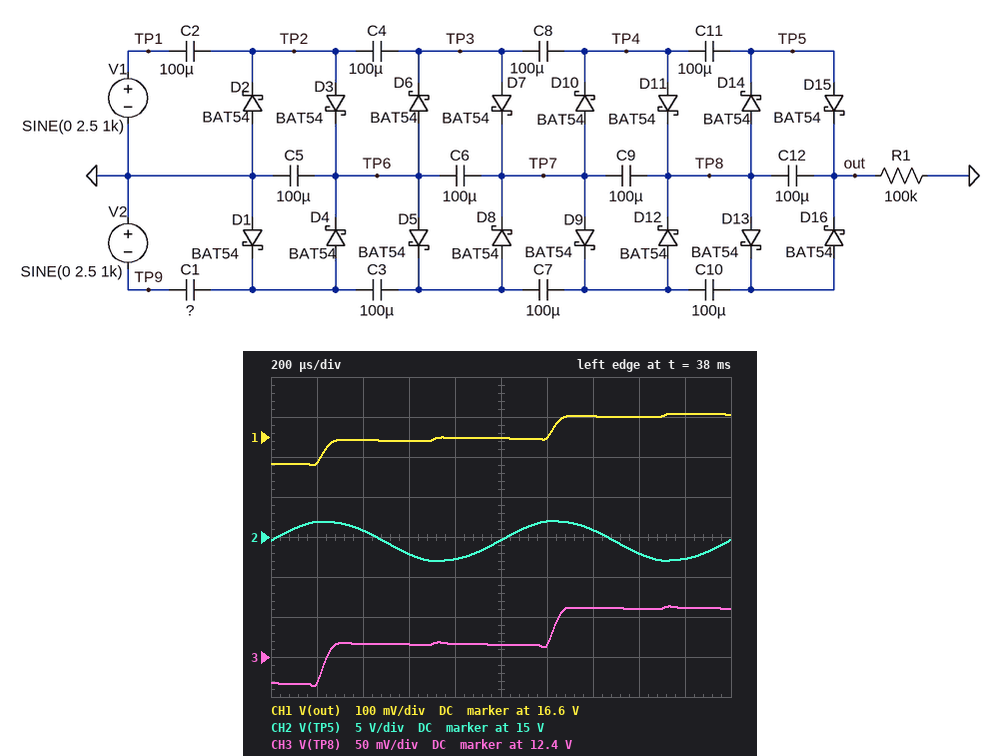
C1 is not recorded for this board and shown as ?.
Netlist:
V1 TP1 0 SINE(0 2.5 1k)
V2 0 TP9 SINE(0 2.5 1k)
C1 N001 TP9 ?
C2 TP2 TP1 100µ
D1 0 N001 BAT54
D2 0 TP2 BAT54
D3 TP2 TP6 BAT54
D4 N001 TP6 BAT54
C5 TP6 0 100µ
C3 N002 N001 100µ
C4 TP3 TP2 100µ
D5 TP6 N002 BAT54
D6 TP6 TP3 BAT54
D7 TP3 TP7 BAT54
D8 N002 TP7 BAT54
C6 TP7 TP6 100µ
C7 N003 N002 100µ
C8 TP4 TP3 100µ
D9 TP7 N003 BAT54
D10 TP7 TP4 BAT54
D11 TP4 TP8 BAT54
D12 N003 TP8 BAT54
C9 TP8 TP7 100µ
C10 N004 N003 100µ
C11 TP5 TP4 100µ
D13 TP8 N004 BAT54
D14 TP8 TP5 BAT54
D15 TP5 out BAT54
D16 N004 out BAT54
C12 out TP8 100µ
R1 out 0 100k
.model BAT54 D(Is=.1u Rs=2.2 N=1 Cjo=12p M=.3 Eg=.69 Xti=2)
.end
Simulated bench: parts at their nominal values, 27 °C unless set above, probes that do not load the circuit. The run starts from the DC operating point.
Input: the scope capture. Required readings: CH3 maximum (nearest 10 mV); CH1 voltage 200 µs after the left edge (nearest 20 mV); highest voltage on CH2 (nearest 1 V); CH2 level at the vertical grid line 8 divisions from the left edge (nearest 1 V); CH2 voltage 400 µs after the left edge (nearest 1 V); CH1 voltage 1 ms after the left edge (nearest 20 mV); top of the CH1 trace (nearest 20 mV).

12.46 V
16.54 V
17 V
13 V
16 V
16.60 V
16.66 V
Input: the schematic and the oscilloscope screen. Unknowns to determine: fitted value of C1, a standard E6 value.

47 µF
